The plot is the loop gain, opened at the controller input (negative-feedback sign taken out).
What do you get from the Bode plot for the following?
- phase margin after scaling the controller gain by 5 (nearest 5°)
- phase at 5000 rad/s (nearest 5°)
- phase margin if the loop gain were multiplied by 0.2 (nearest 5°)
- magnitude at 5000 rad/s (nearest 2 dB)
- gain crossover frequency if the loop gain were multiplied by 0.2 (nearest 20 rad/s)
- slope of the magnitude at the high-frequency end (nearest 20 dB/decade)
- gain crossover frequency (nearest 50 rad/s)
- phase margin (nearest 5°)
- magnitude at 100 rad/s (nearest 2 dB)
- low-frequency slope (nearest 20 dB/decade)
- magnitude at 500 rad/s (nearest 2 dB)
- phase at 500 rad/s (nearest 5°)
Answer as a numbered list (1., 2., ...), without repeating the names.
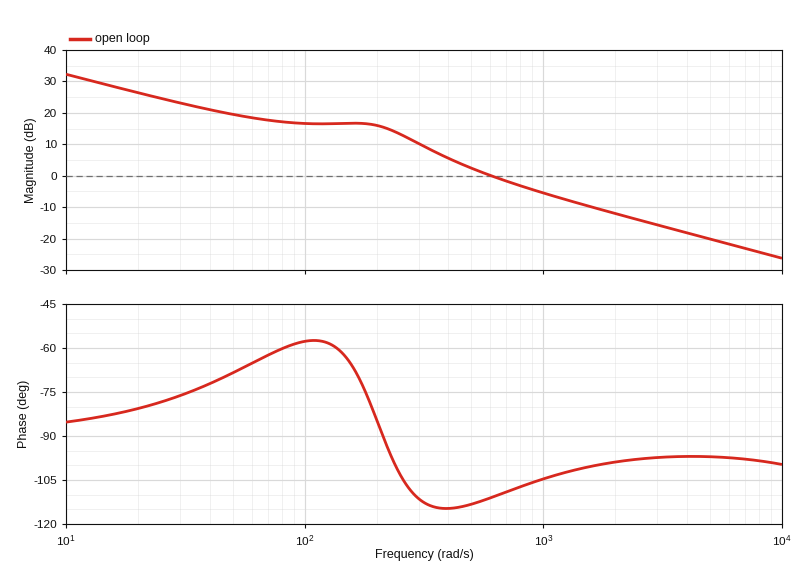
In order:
1. 80°
2. -95°
3. 80°
4. -20 dB
5. 240 rad/s
6. -20 dB/decade
7. 600 rad/s
8. 70°
9. 16 dB
10. -20 dB/decade
11. 2 dB
12. -115°
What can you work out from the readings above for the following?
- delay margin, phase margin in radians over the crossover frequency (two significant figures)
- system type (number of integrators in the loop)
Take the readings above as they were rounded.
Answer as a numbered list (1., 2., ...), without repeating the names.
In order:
1. 0.0020 s
2. 1
